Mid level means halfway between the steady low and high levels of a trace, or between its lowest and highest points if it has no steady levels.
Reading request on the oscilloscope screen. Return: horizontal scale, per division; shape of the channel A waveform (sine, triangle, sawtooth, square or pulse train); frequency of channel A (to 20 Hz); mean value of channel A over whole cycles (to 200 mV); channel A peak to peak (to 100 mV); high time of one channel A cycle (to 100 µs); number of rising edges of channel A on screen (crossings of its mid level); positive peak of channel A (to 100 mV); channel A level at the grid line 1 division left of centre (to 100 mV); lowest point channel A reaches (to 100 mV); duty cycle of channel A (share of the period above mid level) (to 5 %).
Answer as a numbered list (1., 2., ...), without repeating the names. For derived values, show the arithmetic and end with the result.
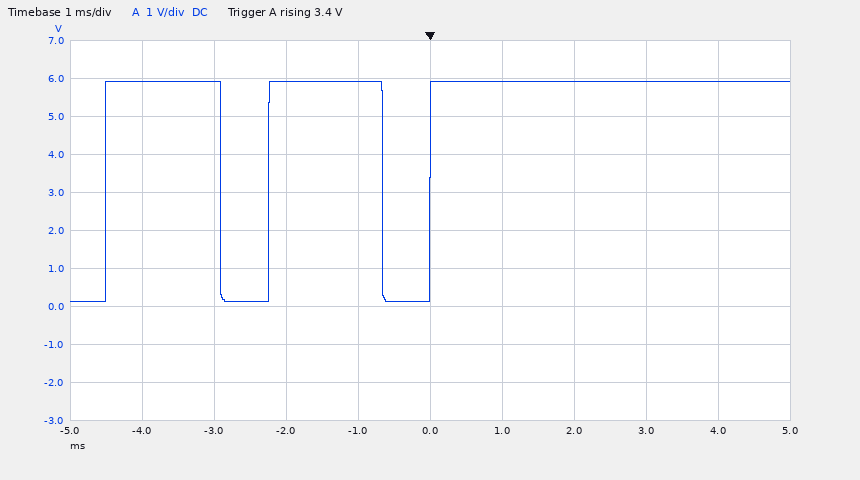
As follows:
1. 1 ms
2. pulse train
3. 440 Hz
4. 100 mV + 0.7 × (5.9 V − (100 mV)) ≈ 4.2 V
5. 5.9 V − (100 mV) = 5.8 V
6. 1.6 ms
7. 3
8. 5.9 V
9. 5.9 V
10. 100 mV
11. 70 %
